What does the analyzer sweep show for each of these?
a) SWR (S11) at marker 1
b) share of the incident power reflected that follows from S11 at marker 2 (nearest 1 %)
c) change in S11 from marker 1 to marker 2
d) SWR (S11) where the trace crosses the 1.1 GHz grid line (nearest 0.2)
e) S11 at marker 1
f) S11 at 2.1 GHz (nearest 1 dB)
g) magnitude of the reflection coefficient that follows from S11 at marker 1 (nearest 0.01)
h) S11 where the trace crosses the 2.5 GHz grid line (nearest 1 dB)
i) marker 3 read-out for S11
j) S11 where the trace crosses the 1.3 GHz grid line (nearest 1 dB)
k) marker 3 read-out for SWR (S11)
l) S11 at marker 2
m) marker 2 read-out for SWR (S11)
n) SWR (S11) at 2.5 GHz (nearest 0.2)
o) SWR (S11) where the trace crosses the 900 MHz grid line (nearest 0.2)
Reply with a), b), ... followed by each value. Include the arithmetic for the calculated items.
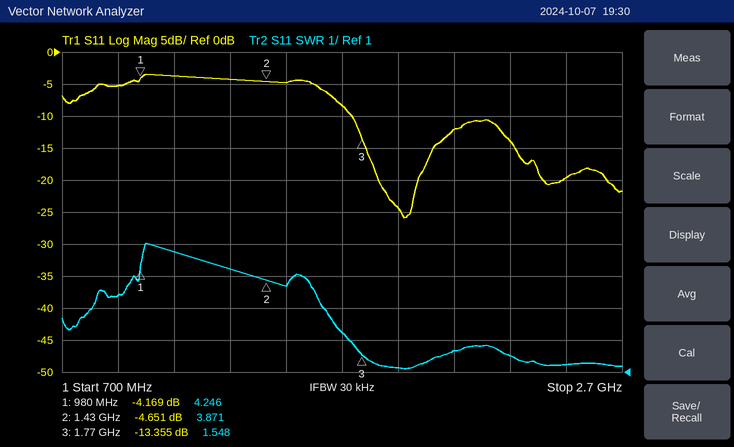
a) 4.246
b) 10^(-4.651/10) ≈ 34 %
c) -4.651 − (-4.169) = -0.482 dB
d) 4.8
e) -4.169 dB
f) -12 dB
g) 10^(-4.169/20) ≈ 0.62
h) -20 dB
i) -13.355 dB
j) -4 dB
k) 1.548
l) -4.651 dB
m) 3.871
n) 1.2
o) 3.4
